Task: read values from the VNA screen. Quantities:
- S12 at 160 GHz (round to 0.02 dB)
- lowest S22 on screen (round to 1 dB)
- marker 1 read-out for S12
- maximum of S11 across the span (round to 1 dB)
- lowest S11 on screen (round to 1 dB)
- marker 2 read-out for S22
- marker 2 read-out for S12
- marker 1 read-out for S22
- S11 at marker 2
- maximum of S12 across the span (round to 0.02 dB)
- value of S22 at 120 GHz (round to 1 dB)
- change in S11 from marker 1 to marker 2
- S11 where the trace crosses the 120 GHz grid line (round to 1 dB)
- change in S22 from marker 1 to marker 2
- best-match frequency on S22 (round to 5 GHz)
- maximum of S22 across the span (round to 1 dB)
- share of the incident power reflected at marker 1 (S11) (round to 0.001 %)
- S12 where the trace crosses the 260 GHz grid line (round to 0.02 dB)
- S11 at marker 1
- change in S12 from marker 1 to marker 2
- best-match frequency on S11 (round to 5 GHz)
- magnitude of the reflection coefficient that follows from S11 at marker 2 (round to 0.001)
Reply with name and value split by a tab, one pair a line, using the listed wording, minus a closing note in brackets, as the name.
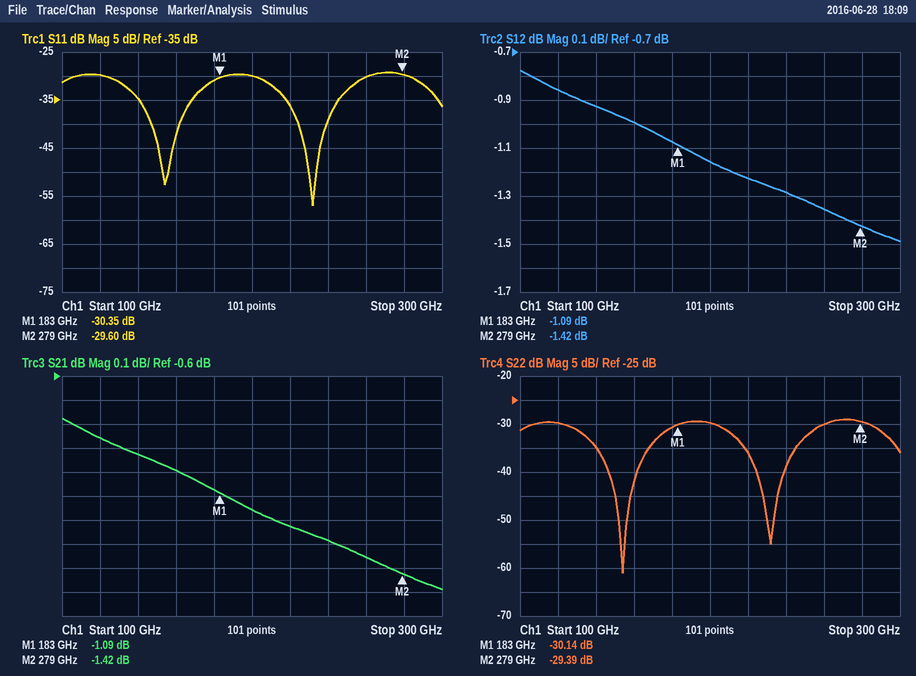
S12 at 160 GHz	-1.00 dB
lowest S22 on screen	-61 dB
marker 1 read-out for S12	-1.09 dB
maximum of S11 across the span	-29 dB
lowest S11 on screen	-57 dB
marker 2 read-out for S22	-29.39 dB
marker 2 read-out for S12	-1.42 dB
marker 1 read-out for S22	-30.14 dB
S11 at marker 2	-29.60 dB
maximum of S12 across the span	-0.78 dB
value of S22 at 120 GHz	-30 dB
change in S11 from marker 1 to marker 2	0.75 dB
S11 where the trace crosses the 120 GHz grid line	-30 dB
change in S22 from marker 1 to marker 2	0.75 dB
best-match frequency on S22	155 GHz
maximum of S22 across the span	-29 dB
share of the incident power reflected at marker 1 (S11)	0.092 %
S12 where the trace crosses the 260 GHz grid line	-1.36 dB
S11 at marker 1	-30.35 dB
change in S12 from marker 1 to marker 2	-0.33 dB
best-match frequency on S11	230 GHz
magnitude of the reflection coefficient that follows from S11 at marker 2	0.033
